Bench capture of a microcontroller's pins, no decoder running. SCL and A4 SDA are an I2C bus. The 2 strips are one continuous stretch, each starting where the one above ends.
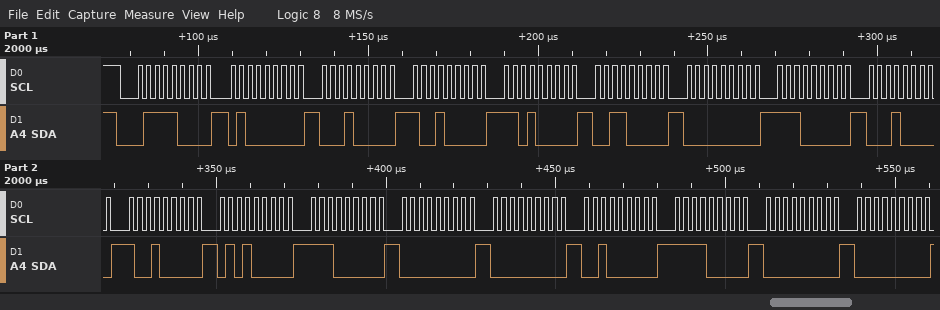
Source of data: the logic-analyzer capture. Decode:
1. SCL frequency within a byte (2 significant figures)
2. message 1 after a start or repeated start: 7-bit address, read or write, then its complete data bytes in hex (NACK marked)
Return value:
400 kHz
0x3C write: 40 10 90 D0 30 00 E0 10 90 50 E0 00 00 20 F0 00 00
